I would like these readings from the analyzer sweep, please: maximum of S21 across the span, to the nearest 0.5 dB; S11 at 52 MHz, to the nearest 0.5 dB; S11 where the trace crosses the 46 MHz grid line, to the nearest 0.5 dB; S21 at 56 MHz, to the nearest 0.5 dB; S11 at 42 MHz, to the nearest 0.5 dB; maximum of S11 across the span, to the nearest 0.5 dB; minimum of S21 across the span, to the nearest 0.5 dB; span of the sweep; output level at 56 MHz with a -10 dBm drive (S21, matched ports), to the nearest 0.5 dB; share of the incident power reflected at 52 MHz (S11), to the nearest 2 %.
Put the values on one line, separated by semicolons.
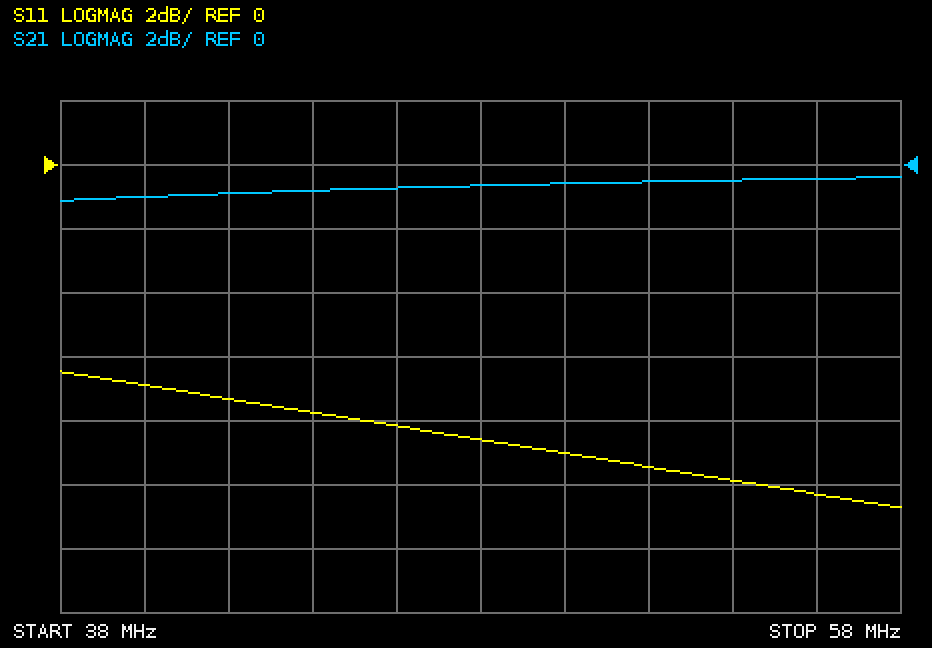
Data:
-0.5 dB; -9.5 dB; -8.0 dB; -0.5 dB; -7.5 dB; -6.5 dB; -1.0 dB; 20 MHz; -10.5 dBm; 12 %
